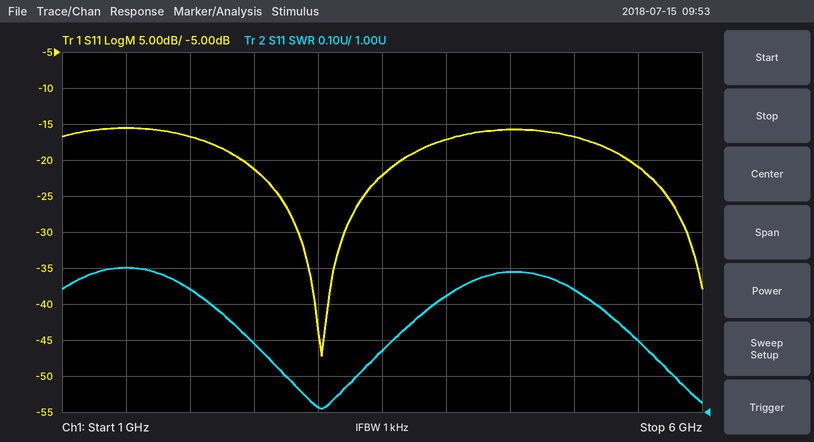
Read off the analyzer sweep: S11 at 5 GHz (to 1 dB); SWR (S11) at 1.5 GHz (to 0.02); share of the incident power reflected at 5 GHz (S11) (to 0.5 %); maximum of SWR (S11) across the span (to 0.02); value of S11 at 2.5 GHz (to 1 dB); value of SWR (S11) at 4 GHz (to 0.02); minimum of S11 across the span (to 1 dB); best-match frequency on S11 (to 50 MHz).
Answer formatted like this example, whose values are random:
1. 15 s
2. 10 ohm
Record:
1. -17 dB
2. 1.40
3. 2.0 %
4. 1.40
5. -21 dB
6. 1.32
7. -47 dB
8. 3.05 GHz
